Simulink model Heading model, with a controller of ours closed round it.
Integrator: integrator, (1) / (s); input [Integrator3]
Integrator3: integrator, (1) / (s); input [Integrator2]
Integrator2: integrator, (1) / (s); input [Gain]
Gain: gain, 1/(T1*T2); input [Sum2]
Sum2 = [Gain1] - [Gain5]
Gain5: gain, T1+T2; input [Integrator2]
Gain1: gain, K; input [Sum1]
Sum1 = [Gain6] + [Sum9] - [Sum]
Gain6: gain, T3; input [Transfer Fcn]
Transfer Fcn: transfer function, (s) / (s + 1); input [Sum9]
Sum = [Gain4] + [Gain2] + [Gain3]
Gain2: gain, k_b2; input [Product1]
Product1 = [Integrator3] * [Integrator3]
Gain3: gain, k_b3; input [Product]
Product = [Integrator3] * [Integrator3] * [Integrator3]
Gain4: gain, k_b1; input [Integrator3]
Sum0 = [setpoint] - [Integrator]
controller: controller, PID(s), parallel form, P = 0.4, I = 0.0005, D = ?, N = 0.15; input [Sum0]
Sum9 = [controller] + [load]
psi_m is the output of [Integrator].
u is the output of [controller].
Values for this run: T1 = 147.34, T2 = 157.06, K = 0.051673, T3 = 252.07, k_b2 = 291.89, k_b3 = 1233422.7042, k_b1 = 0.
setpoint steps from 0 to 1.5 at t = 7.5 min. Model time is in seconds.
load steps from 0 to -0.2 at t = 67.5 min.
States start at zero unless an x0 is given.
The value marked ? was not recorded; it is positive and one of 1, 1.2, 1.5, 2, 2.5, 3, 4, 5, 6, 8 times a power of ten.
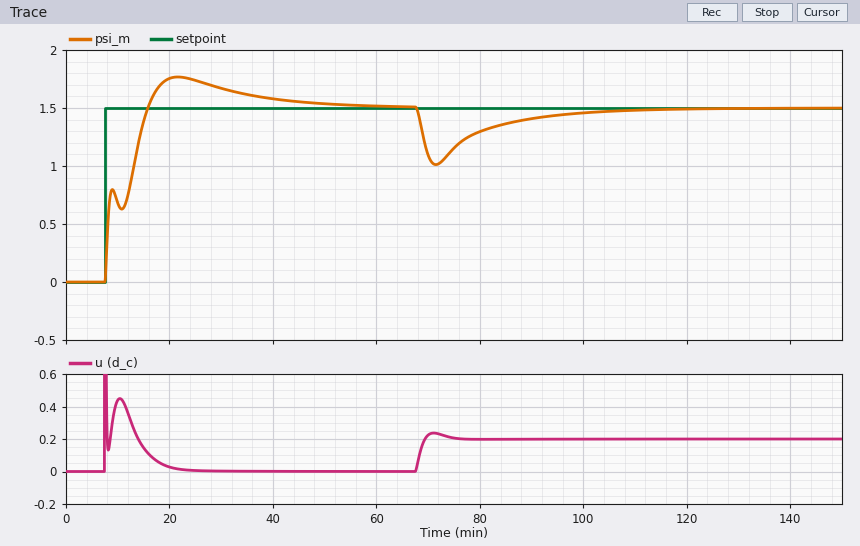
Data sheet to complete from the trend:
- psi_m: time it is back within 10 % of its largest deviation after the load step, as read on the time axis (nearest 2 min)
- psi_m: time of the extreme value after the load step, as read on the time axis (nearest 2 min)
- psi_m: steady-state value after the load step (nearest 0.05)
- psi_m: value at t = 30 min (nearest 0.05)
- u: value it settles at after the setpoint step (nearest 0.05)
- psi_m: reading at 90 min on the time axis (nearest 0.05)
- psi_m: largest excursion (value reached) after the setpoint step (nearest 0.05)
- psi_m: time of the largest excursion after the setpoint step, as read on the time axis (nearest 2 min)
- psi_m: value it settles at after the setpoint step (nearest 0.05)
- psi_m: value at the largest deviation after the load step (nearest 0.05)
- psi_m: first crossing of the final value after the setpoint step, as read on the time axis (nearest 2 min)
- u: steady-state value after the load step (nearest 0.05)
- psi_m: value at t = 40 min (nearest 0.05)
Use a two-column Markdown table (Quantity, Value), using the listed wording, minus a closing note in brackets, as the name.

| Quantity | Value |
|---|---|
| psi_m: time it is back within 10 % of its largest deviation after the load step, as read on the time axis | 98 min |
| psi_m: time of the extreme value after the load step, as read on the time axis | 72 min |
| psi_m: steady-state value after the load step | 1.50 |
| psi_m: value at t = 30 min | 1.65 |
| u: value it settles at after the setpoint step | 0.00 |
| psi_m: reading at 90 min on the time axis | 1.40 |
| psi_m: largest excursion (value reached) after the setpoint step | 1.75 |
| psi_m: time of the largest excursion after the setpoint step, as read on the time axis | 22 min |
| psi_m: value it settles at after the setpoint step | 1.50 |
| psi_m: value at the largest deviation after the load step | 1.00 |
| psi_m: first crossing of the final value after the setpoint step, as read on the time axis | 16 min |
| u: steady-state value after the load step | 0.20 |
| psi_m: value at t = 40 min | 1.60 |
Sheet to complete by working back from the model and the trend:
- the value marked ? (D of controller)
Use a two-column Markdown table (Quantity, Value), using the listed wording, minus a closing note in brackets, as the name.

| Quantity | Value |
|---|---|
| the value marked ? | 20 |
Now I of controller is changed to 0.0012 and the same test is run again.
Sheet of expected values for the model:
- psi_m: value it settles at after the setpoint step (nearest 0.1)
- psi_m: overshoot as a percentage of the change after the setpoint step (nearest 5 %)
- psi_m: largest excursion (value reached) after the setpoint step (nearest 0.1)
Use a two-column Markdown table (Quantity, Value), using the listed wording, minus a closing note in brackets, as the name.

| Quantity | Value |
|---|---|
| psi_m: value it settles at after the setpoint step | 1.5 |
| psi_m: overshoot as a percentage of the change after the setpoint step | 25 % |
| psi_m: largest excursion (value reached) after the setpoint step | 1.9 |
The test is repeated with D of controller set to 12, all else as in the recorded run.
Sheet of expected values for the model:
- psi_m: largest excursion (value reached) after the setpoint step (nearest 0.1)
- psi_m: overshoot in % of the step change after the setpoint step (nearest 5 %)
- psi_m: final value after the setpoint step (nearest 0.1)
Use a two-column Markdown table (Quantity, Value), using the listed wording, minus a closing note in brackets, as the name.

| Quantity | Value |
|---|---|
| psi_m: largest excursion (value reached) after the setpoint step | 1.7 |
| psi_m: overshoot in % of the step change after the setpoint step | 15 % |
| psi_m: final value after the setpoint step | 1.5 |
